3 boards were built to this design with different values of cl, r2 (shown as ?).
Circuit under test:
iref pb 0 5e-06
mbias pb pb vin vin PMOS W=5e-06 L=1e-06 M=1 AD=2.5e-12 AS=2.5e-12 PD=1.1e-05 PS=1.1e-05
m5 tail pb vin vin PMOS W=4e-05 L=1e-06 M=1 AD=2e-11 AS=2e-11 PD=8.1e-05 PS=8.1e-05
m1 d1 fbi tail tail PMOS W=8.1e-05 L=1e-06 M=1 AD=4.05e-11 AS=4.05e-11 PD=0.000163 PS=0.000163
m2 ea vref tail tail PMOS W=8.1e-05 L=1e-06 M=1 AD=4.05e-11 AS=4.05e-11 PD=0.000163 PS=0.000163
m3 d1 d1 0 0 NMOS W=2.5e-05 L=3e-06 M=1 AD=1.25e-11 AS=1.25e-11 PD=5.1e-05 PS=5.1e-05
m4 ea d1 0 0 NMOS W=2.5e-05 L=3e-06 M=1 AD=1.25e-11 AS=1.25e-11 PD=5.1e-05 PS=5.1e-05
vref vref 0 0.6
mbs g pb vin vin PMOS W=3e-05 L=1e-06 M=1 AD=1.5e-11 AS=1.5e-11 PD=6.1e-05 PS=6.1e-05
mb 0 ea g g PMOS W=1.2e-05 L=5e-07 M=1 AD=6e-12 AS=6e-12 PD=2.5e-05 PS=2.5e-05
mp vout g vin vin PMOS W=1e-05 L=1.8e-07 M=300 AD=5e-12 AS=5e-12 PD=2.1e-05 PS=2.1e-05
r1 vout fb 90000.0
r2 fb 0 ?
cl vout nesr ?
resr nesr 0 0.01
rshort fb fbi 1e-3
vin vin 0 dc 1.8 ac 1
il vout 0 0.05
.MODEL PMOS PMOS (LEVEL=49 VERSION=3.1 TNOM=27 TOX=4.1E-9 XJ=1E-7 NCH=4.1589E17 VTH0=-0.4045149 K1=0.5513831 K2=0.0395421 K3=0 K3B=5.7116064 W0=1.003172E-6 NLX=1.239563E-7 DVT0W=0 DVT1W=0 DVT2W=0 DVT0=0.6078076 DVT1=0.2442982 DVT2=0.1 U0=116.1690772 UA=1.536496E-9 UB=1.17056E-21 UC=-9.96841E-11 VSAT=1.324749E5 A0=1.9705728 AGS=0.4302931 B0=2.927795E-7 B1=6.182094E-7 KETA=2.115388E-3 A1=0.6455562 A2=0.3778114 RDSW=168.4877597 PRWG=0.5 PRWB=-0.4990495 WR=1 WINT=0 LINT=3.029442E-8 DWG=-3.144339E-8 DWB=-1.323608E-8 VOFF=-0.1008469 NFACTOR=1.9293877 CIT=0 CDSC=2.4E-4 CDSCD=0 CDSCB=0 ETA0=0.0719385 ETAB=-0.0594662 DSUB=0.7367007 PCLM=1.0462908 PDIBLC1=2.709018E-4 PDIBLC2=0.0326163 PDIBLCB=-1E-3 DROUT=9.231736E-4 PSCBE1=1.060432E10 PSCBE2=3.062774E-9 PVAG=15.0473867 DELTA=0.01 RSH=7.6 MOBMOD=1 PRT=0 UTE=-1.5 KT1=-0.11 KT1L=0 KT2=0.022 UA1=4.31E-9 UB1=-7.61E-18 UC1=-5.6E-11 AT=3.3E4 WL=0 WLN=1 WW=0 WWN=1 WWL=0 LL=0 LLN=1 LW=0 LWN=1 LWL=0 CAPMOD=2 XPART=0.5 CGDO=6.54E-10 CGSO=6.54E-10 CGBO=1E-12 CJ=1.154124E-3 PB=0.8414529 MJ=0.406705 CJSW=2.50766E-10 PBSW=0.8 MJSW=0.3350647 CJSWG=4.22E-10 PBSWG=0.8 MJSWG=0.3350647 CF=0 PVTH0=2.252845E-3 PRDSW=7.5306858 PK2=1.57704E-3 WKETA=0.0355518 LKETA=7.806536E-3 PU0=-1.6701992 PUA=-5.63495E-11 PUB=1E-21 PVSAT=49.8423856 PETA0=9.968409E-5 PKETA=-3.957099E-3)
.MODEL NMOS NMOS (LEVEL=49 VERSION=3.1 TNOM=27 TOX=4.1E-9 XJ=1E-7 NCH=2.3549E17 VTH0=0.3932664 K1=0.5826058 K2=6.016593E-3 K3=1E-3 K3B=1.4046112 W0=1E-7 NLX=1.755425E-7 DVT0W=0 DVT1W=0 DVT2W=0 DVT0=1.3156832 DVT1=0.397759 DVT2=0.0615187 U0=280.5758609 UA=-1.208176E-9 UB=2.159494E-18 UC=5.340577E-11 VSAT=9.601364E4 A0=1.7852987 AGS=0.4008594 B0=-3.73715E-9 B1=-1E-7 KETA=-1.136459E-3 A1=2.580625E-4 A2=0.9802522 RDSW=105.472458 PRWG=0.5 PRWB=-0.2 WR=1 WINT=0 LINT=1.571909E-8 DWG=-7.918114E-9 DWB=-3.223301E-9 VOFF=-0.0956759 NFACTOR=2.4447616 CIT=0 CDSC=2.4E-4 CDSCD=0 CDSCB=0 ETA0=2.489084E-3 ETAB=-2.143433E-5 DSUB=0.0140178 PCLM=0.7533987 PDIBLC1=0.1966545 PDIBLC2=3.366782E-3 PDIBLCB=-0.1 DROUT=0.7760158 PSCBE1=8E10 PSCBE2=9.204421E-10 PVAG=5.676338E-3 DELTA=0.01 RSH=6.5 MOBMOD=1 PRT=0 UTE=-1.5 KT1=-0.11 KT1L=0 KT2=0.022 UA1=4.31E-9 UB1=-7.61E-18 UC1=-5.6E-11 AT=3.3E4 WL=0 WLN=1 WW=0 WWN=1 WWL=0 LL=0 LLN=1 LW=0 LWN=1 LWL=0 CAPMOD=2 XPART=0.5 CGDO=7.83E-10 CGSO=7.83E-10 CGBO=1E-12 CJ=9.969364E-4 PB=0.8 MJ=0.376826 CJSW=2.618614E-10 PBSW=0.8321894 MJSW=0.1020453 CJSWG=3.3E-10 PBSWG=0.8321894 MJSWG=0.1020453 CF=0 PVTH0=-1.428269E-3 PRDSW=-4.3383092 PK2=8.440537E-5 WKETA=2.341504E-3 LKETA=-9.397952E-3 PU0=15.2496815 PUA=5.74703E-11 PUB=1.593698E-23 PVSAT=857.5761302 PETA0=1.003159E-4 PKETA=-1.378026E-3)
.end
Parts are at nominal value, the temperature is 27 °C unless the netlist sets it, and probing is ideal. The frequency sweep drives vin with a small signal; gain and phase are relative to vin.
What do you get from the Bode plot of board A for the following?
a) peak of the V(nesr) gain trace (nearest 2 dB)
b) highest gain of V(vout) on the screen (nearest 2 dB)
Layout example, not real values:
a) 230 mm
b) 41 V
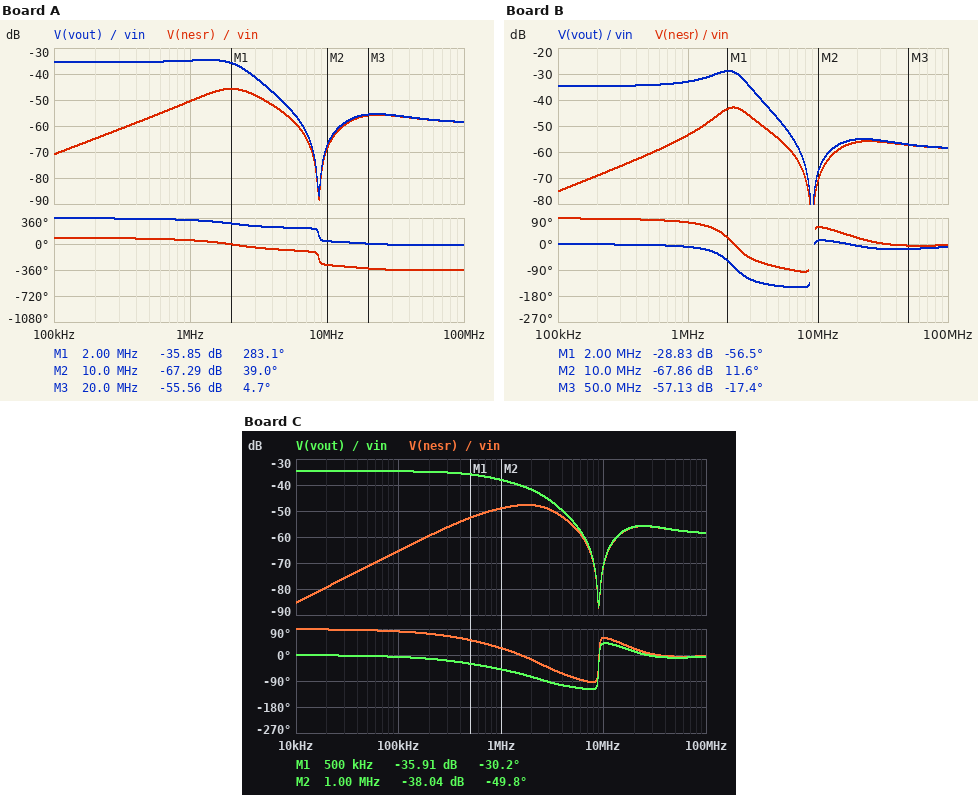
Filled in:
a) -46 dB
b) -34 dB
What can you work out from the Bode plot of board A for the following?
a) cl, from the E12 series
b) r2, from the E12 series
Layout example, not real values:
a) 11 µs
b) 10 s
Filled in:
a) 2.7 µF
b) 150 kΩ
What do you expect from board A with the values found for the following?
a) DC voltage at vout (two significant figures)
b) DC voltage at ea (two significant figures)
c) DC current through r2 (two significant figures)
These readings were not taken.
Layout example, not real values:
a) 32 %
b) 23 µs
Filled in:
a) 960 mV
b) 400 mV
c) 4.0 µA
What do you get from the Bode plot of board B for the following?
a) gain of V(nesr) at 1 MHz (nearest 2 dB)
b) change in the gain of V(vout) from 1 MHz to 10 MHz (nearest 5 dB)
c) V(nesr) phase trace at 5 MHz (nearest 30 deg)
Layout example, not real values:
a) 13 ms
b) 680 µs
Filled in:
a) -54 dB
b) -35 dB
c) -90 deg
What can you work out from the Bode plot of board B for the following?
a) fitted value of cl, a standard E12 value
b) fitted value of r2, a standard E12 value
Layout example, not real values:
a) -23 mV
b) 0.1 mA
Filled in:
a) 1.5 µF
b) 120 kΩ
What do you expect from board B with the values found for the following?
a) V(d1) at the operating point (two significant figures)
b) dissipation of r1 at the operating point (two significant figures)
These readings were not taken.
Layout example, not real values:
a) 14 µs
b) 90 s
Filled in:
a) 560 mV
b) 2.2 µW
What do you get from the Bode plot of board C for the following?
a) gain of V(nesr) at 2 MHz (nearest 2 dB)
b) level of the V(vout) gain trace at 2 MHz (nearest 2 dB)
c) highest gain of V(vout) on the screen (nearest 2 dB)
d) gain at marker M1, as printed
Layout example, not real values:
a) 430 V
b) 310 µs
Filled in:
a) -48 dB
b) -42 dB
c) -34 dB
d) -35.91 dB
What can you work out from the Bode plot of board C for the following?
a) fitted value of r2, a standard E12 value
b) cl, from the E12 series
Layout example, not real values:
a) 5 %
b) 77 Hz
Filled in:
a) 120 kΩ
b) 4.7 µF
